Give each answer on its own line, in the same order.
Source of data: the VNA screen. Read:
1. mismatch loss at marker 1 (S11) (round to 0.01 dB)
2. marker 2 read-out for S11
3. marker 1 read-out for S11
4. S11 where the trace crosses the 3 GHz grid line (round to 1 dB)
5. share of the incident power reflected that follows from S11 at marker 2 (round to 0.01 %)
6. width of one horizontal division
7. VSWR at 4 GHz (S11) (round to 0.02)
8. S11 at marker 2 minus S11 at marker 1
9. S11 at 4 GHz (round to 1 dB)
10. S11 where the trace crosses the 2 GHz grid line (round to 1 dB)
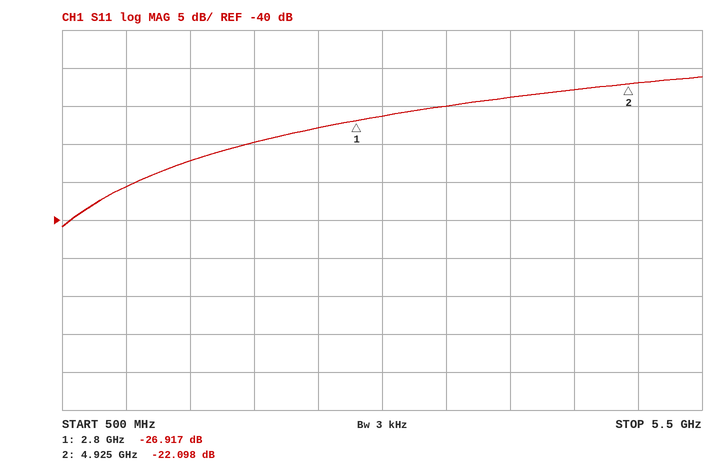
0.01 dB
-22.098 dB
-26.917 dB
-26 dB
0.62 %
500 MHz
1.14
4.819 dB
-24 dB
-30 dB
